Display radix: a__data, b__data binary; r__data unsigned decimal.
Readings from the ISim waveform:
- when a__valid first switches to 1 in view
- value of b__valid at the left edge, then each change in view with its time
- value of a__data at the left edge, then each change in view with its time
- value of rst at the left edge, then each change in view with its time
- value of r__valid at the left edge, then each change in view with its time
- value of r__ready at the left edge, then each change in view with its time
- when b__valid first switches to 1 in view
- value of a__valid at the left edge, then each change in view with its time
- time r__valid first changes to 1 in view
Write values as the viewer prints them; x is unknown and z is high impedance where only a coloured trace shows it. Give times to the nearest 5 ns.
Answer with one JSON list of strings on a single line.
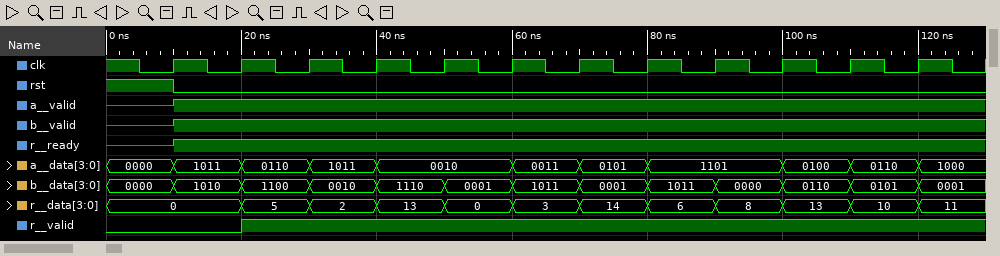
["10 ns", "z, 1 at 10 ns", "0000, 1011 at 10 ns, 0110 at 20 ns, 1011 at 30 ns, 0010 at 40 ns, 0011 at 60 ns, 0101 at 70 ns, 1101 at 80 ns, 0100 at 100 ns, 0110 at 110 ns, 1000 at 120 ns", "1, 0 at 10 ns", "0, 1 at 20 ns", "z, 1 at 10 ns", "10 ns", "z, 1 at 10 ns", "20 ns"]
